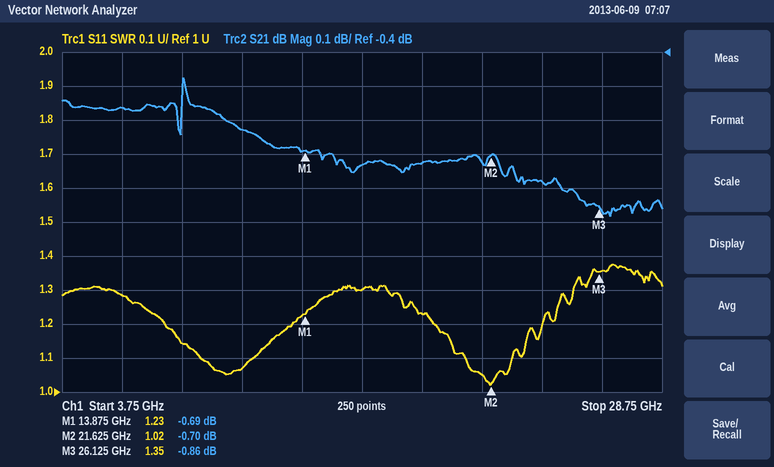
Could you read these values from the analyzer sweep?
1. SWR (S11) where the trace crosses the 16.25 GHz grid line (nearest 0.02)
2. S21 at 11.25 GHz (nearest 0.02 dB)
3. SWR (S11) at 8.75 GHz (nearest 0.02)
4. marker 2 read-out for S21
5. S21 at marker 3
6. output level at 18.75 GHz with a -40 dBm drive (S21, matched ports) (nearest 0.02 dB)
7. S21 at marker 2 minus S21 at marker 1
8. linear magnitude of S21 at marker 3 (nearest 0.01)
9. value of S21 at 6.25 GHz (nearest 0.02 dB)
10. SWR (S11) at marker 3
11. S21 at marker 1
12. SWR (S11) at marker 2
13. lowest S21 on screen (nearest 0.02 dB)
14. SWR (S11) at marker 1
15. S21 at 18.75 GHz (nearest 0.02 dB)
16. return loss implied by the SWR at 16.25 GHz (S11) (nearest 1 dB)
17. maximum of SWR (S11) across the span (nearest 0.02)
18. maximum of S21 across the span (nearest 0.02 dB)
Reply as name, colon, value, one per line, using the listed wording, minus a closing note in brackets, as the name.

SWR (S11) where the trace crosses the 16.25 GHz grid line: 1.30
S21 at 11.25 GHz: -0.62 dB
SWR (S11) at 8.75 GHz: 1.14
marker 2 read-out for S21: -0.70 dB
S21 at marker 3: -0.86 dB
output level at 18.75 GHz with a -40 dBm drive (S21, matched ports): -40.72 dBm
S21 at marker 2 minus S21 at marker 1: -0.01 dB
linear magnitude of S21 at marker 3: 0.91
value of S21 at 6.25 GHz: -0.56 dB
SWR (S11) at marker 3: 1.35
S21 at marker 1: -0.69 dB
SWR (S11) at marker 2: 1.02
lowest S21 on screen: -0.88 dB
SWR (S11) at marker 1: 1.23
S21 at 18.75 GHz: -0.72 dB
return loss implied by the SWR at 16.25 GHz (S11): 18 dB
maximum of SWR (S11) across the span: 1.38
maximum of S21 across the span: -0.48 dB
